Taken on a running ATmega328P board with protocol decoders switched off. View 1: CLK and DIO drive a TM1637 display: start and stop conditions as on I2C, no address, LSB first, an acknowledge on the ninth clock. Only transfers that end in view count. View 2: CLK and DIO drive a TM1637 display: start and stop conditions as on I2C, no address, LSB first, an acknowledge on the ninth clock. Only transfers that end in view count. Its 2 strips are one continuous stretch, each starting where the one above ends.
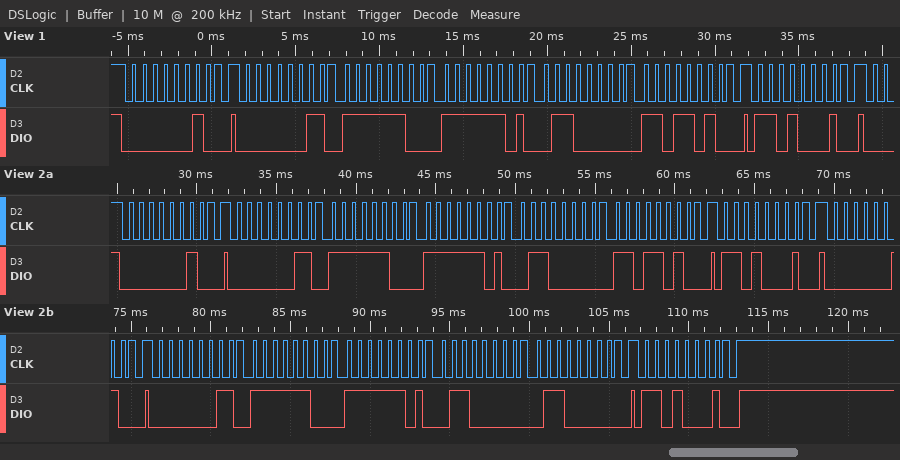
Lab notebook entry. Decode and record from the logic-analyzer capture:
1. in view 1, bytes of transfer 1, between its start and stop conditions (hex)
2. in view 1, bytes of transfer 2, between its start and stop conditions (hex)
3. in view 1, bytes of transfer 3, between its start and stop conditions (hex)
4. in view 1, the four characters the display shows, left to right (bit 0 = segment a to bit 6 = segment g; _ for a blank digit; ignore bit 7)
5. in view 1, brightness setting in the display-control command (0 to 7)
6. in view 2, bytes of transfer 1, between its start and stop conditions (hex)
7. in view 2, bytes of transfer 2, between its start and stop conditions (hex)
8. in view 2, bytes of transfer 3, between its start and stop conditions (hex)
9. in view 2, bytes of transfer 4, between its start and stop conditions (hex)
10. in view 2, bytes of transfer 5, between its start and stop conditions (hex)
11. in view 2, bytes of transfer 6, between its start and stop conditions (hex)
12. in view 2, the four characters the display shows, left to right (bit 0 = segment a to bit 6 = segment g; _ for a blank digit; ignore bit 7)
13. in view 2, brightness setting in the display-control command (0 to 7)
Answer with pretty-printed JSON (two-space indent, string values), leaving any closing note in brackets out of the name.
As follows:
{
  "in view 1, bytes of transfer 1, between its start and stop conditions": "40",
  "in view 1, bytes of transfer 2, between its start and stop conditions": "C0 3F BF 06 5B",
  "in view 1, bytes of transfer 3, between its start and stop conditions": "8B",
  "in view 1, the four characters the display shows, left to right": "0012",
  "in view 1, brightness setting in the display-control command": "3",
  "in view 2, bytes of transfer 1, between its start and stop conditions": "40",
  "in view 2, bytes of transfer 2, between its start and stop conditions": "C0 3F BF 06 5B",
  "in view 2, bytes of transfer 3, between its start and stop conditions": "8B",
  "in view 2, bytes of transfer 4, between its start and stop conditions": "40",
  "in view 2, bytes of transfer 5, between its start and stop conditions": "C0 3F BF 06 06",
  "in view 2, bytes of transfer 6, between its start and stop conditions": "8B",
  "in view 2, the four characters the display shows, left to right": "0011",
  "in view 2, brightness setting in the display-control command": "3"
}
